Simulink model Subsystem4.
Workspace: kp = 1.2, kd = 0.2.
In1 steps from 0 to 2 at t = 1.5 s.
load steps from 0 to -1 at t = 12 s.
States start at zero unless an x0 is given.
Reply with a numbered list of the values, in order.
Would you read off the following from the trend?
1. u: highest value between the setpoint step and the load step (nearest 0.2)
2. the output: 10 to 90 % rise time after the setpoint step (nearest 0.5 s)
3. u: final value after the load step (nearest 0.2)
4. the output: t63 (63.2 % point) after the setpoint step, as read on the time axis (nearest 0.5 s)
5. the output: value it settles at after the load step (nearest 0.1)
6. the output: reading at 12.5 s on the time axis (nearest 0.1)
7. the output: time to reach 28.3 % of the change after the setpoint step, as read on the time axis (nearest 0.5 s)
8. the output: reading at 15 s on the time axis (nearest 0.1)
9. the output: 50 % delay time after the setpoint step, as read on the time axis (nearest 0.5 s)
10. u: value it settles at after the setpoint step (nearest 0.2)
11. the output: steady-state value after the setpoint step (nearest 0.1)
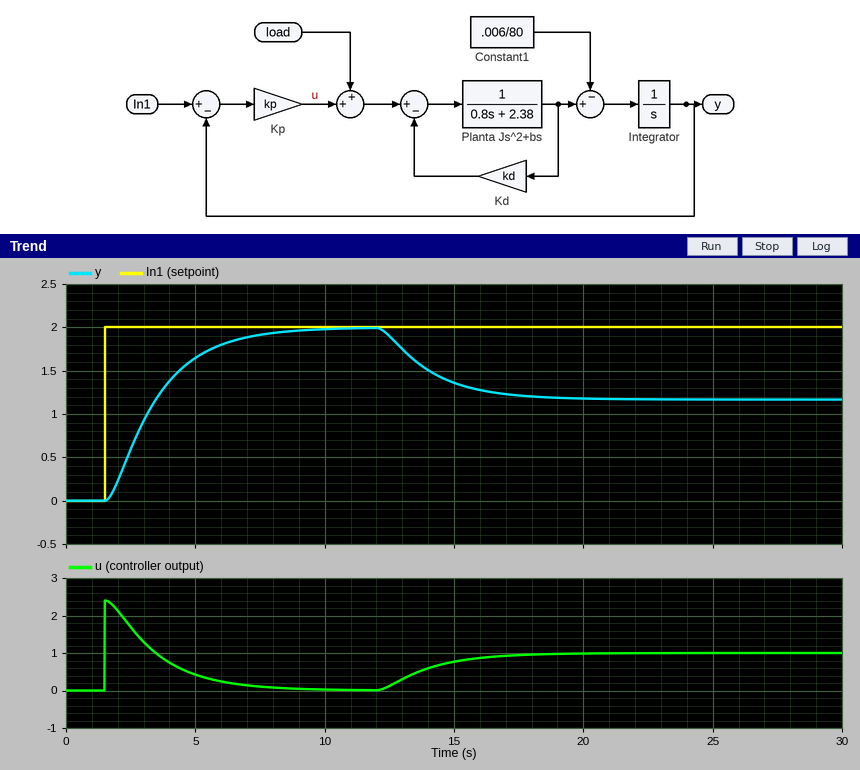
1. 2.4
2. 4.0 s
3. 1.0
4. 3.5 s
5. 1.2
6. 1.9
7. 2.5 s
8. 1.4
9. 3.0 s
10. 0.0
11. 2.0
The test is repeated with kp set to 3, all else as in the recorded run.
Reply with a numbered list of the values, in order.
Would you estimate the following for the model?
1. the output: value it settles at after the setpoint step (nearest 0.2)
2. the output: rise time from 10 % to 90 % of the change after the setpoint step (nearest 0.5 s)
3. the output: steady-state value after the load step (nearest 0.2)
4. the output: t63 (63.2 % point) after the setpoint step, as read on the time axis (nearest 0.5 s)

1. 2.0
2. 1.5 s
3. 1.6
4. 2.5 s
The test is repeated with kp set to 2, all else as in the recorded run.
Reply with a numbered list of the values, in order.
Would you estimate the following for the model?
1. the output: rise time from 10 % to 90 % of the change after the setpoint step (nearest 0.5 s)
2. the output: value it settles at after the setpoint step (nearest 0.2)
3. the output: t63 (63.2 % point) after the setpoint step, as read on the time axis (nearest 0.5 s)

1. 2.0 s
2. 2.0
3. 3.0 s
